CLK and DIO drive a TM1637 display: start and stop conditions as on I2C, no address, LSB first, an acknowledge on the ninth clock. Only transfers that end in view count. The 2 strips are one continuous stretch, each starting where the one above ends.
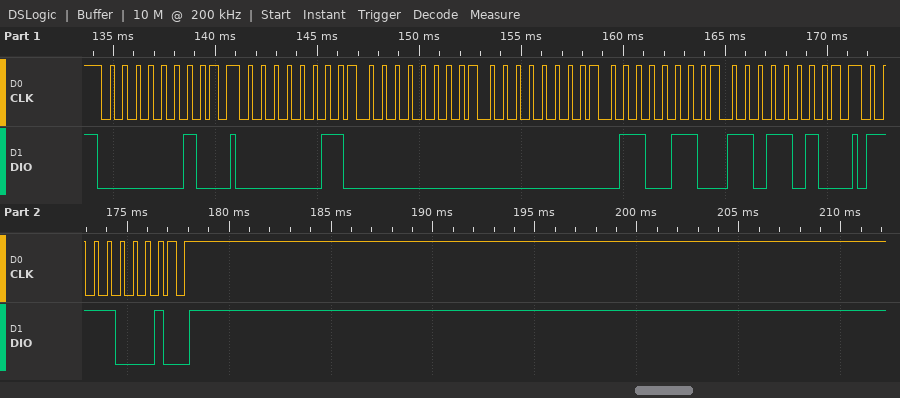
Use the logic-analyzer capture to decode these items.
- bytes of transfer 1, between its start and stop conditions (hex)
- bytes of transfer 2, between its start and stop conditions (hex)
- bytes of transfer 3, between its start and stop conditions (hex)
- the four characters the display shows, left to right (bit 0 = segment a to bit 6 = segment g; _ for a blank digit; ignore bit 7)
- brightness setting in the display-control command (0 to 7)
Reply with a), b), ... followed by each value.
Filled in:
a) 40
b) C0 00 00 66 5B
c) 8F
d) __42
e) 7
